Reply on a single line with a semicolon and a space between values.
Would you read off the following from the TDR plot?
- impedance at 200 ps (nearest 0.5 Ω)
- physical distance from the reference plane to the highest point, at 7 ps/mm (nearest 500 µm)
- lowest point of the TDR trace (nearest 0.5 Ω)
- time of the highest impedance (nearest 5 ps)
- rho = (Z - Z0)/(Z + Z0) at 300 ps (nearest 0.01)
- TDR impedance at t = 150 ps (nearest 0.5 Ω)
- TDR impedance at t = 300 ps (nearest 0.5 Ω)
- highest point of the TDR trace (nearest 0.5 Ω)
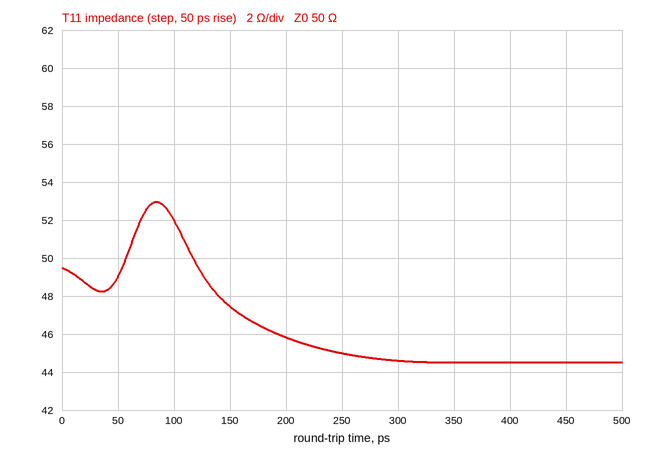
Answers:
46.0 Ω; 6.0 mm; 44.5 Ω; 85 ps; -0.06; 47.5 Ω; 44.5 Ω; 53.0 Ω
